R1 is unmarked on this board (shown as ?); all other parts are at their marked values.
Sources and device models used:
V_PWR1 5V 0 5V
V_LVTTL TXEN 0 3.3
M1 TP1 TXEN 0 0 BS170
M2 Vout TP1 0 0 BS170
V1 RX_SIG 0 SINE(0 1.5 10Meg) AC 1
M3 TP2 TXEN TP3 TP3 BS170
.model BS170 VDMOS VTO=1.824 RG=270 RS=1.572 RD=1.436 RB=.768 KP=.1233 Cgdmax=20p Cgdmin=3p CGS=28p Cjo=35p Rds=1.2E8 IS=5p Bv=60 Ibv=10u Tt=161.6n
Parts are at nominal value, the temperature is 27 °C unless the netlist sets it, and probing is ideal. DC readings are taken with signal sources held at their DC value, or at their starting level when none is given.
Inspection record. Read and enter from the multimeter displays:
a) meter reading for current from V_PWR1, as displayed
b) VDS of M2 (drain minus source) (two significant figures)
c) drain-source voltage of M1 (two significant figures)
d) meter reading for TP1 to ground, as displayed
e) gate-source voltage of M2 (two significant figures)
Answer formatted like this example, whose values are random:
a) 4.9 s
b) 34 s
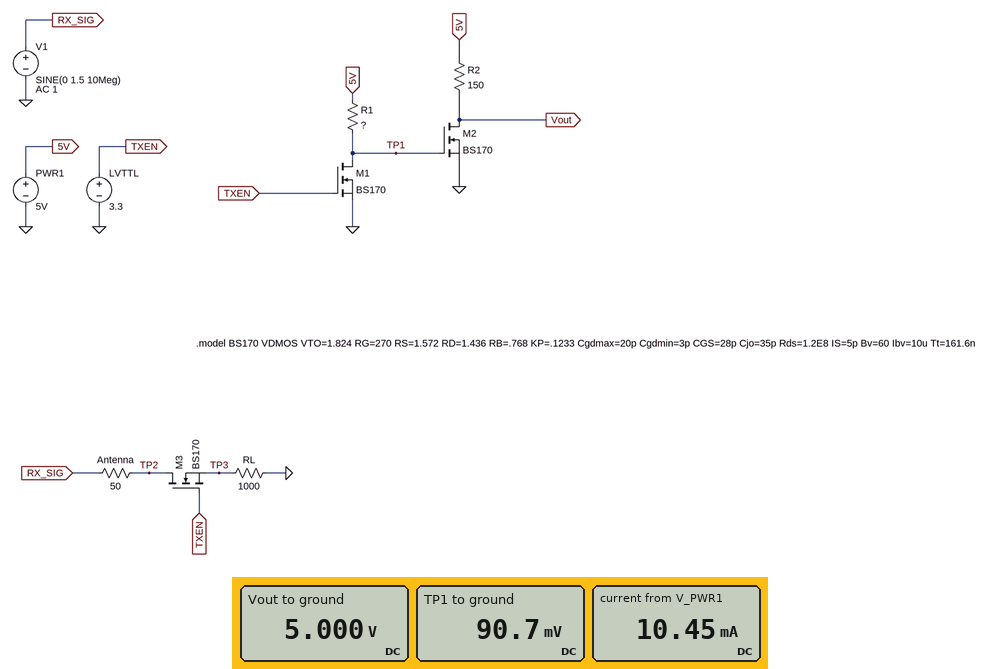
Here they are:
a) 10.45 mA
b) 5.0 V
c) 91 mV
d) 90.7 mV
e) 91 mV
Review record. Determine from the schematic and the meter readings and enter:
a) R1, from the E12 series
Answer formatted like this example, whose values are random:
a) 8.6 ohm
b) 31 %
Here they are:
a) 470 Ω
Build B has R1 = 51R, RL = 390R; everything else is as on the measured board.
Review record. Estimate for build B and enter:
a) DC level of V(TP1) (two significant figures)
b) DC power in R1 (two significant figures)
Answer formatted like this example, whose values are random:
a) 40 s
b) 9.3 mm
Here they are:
a) 880 mV
b) 330 mW
